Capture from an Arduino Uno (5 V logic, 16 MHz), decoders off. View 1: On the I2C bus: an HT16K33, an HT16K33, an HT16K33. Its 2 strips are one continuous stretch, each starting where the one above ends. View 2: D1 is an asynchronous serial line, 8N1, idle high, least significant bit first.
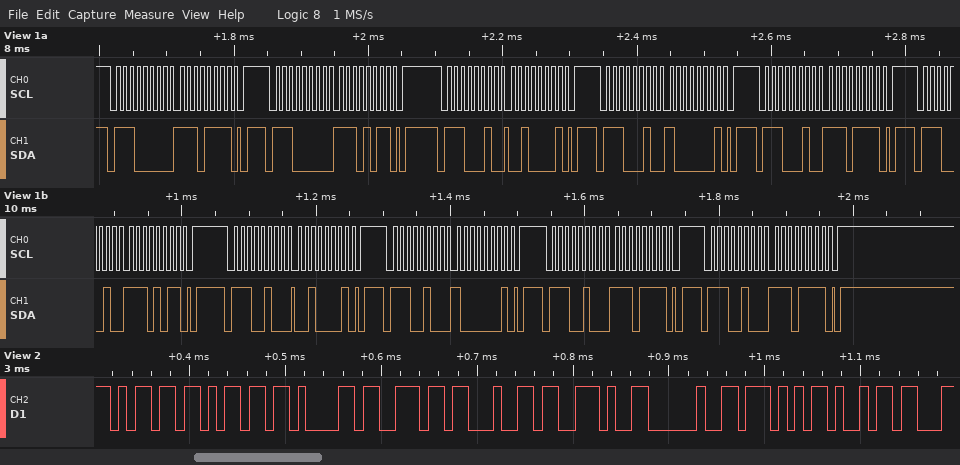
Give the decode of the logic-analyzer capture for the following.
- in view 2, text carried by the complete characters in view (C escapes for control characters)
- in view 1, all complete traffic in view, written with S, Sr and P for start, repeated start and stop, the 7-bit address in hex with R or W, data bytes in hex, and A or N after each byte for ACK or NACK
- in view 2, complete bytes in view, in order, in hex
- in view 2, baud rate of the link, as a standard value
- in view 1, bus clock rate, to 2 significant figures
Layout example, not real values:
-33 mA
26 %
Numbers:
"mmand. Wi"
S 70W A EF A P S 70W A EB A P S 71W A 21 A P S 71W A 81 A P S 71W A EF A P S 71W A EB A P S 72W A 21 A P S 72W A 81 A P S 72W A EF A P S 72W A EF A P
6D 6D 61 6E 64 2E 20 57 69
115200 baud
100 kHz
